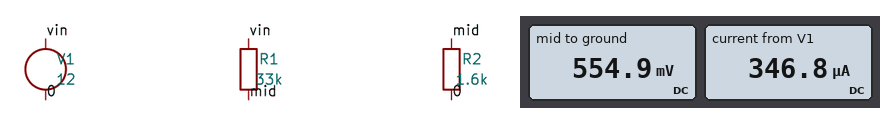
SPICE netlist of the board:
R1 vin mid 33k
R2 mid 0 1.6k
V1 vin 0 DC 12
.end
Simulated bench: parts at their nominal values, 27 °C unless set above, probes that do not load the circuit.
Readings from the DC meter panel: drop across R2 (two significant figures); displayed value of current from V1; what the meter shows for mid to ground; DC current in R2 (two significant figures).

550 mV
346.8 µA
554.9 mV
350 µA
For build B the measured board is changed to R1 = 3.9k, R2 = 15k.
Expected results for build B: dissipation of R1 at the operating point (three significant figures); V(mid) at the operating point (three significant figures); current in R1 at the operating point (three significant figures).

1.57 mW
9.52 V
635 µA
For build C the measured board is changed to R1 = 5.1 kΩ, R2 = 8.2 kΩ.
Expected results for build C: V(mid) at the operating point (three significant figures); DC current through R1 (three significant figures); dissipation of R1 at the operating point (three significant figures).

7.40 V
902 µA
4.15 mW
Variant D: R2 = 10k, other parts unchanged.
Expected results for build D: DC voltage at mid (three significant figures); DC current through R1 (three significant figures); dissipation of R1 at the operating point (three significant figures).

2.79 V
279 µA
2.57 mW
